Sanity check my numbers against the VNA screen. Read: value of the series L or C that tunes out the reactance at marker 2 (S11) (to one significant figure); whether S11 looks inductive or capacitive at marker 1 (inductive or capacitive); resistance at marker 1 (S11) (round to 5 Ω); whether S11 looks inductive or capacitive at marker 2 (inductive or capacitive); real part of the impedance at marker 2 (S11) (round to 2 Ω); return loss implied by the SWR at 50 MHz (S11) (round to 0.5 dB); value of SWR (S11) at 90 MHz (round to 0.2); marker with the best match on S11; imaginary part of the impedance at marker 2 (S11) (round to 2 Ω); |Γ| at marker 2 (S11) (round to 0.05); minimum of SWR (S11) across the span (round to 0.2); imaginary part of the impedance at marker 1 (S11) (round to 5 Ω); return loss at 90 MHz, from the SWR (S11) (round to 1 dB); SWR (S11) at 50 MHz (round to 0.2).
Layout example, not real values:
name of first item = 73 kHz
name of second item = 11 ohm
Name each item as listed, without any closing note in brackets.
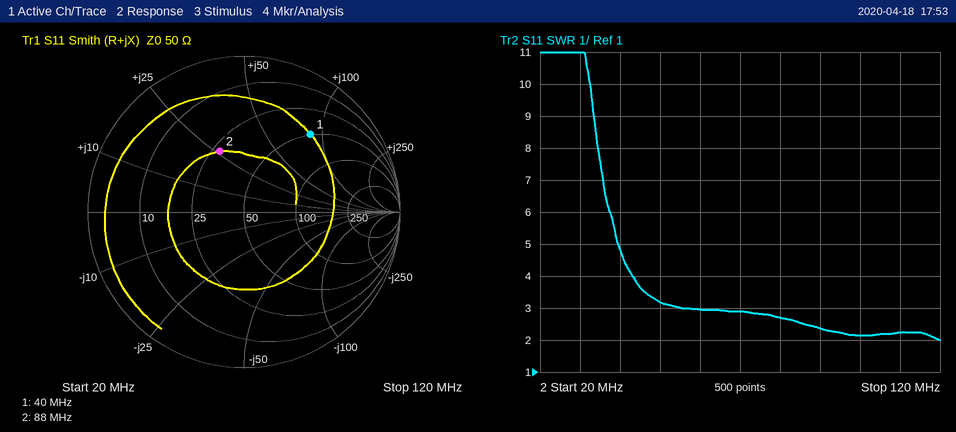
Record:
value of the series L or C that tunes out the reactance at marker 2 (S11) = 70 pF
whether S11 looks inductive or capacitive at marker 1 = inductive
resistance at marker 1 (S11) = 50 Ω
whether S11 looks inductive or capacitive at marker 2 = inductive
real part of the impedance at marker 2 (S11) = 28 Ω
return loss implied by the SWR at 50 MHz (S11) = 5.5 dB
value of SWR (S11) at 90 MHz = 2.4
marker with the best match on S11 = marker 2
imaginary part of the impedance at marker 2 (S11) = +26 Ω
|Γ| at marker 2 (S11) = 0.40
minimum of SWR (S11) across the span = 2.0
imaginary part of the impedance at marker 1 (S11) = +85 Ω
return loss at 90 MHz, from the SWR (S11) = 8 dB
SWR (S11) at 50 MHz = 3.2
